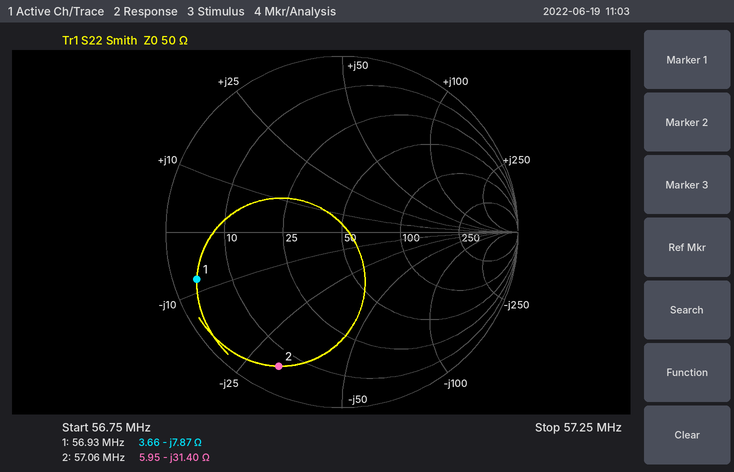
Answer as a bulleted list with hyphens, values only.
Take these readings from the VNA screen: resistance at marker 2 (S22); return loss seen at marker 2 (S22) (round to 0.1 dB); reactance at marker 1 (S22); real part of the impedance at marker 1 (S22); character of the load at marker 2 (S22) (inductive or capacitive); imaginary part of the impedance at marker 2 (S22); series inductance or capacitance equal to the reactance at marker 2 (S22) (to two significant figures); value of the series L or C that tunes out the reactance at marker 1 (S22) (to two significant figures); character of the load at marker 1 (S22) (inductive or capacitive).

- 5.95 Ω
- 1.5 dB
- -7.87 Ω
- 3.66 Ω
- capacitive
- -31.40 Ω
- 89 pF
- 22 nH
- capacitive
